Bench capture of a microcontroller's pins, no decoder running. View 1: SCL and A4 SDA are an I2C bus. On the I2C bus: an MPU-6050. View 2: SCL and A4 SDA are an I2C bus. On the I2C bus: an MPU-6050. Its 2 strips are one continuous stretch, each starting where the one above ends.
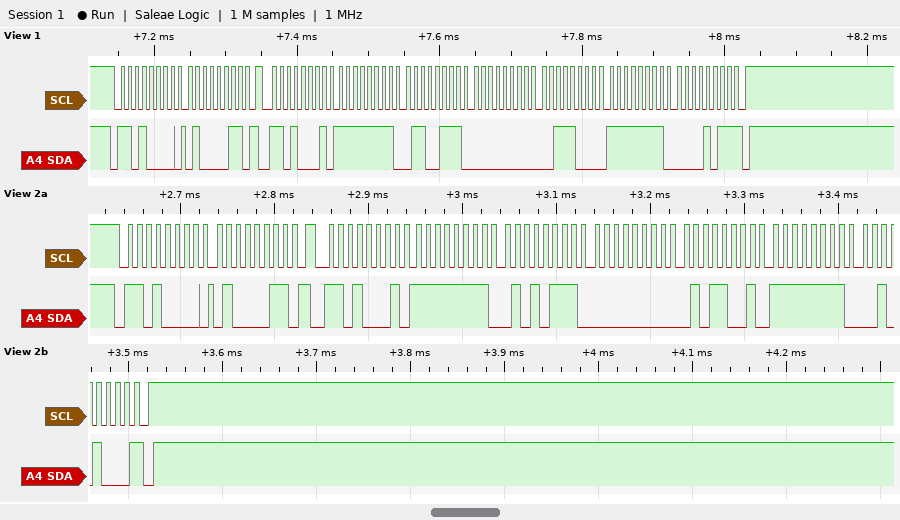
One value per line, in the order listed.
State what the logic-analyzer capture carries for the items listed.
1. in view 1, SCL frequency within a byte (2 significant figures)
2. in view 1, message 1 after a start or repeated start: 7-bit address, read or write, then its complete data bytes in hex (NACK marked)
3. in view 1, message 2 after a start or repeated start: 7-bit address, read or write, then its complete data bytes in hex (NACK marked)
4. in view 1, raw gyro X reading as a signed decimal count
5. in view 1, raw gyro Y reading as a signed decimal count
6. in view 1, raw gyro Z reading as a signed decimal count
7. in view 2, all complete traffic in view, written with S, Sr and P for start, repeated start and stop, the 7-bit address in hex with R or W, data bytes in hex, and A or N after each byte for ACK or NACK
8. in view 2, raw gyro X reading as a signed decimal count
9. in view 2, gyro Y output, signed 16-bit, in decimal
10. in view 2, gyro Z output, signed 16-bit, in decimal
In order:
100 kHz
0x68 write: 43
0x68 read: FF 67 00 38 FF 0B NACK
-153
56
-245
S 68W A 43 A Sr 68R A FF A 57 A 00 A 59 A FF A 28 N P
-169
89
-216
